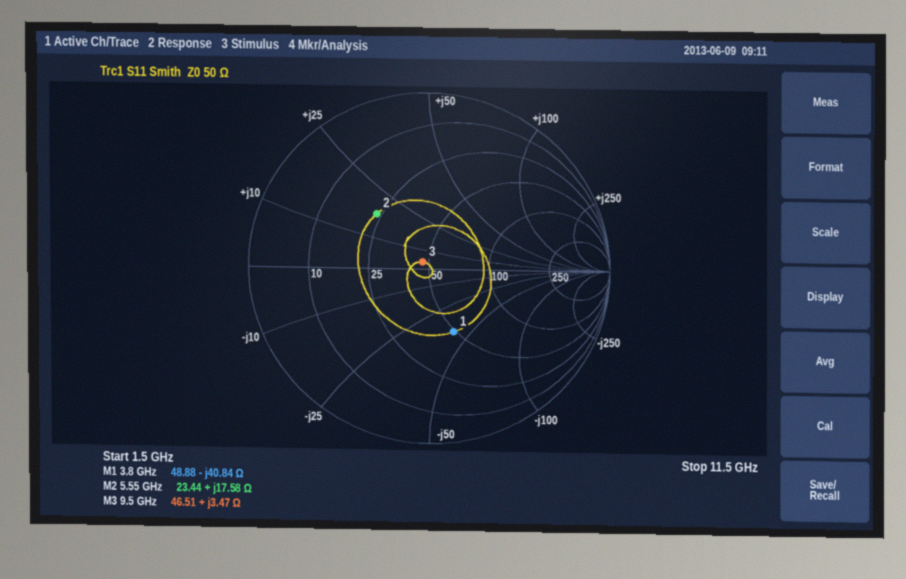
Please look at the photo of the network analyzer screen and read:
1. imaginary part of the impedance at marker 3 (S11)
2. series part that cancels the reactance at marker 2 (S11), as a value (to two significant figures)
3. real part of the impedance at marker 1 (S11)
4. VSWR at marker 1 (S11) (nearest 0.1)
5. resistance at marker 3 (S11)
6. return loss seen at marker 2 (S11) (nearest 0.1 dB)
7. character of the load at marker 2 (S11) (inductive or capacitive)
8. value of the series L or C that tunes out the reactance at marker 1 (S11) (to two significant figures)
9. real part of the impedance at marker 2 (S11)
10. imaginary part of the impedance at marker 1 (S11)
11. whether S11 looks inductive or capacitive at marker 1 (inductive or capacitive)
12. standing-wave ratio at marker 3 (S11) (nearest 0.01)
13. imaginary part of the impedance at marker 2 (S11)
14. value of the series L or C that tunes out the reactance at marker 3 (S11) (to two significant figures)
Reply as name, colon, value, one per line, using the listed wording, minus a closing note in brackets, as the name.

imaginary part of the impedance at marker 3: +3.47 Ω
series part that cancels the reactance at marker 2 (S11), as a value: 1.6 pF
real part of the impedance at marker 1: 48.88 Ω
VSWR at marker 1 (S11): 2.2
resistance at marker 3: 46.51 Ω
return loss seen at marker 2 (S11): 7.5 dB
character of the load at marker 2 (S11): inductive
value of the series L or C that tunes out the reactance at marker 1 (S11): 1.7 nH
real part of the impedance at marker 2: 23.44 Ω
imaginary part of the impedance at marker 1: -40.84 Ω
whether S11 looks inductive or capacitive at marker 1: capacitive
standing-wave ratio at marker 3 (S11): 1.11
imaginary part of the impedance at marker 2: +17.58 Ω
value of the series L or C that tunes out the reactance at marker 3 (S11): 4.8 pF
